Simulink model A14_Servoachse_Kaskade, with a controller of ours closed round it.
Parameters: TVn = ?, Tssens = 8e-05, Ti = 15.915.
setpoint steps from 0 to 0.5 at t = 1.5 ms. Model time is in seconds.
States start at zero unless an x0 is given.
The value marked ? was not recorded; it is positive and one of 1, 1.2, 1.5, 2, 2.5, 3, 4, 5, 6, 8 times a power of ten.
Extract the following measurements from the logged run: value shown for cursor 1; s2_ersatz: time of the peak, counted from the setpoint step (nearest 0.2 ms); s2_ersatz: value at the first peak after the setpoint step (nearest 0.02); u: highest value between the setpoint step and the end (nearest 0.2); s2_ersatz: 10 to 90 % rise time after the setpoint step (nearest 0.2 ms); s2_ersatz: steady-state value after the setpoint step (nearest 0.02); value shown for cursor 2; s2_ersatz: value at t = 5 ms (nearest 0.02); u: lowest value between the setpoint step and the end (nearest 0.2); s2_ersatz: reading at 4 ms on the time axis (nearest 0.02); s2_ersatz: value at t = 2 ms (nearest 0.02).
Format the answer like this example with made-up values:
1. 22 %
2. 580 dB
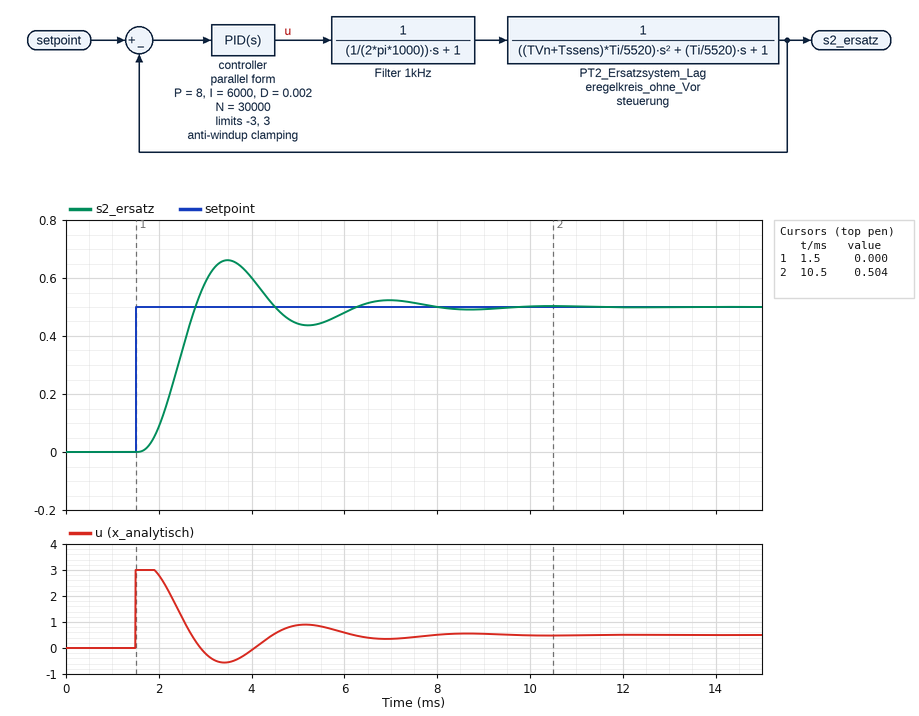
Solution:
1. 0.000
2. 2.0 ms
3. 0.66
4. 3.0
5. 0.8 ms
6. 0.50
7. 0.504
8. 0.44
9. -0.6
10. 0.60
11. 0.08
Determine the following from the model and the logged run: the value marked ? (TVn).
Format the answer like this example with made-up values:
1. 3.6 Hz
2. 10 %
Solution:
1. 0.0006
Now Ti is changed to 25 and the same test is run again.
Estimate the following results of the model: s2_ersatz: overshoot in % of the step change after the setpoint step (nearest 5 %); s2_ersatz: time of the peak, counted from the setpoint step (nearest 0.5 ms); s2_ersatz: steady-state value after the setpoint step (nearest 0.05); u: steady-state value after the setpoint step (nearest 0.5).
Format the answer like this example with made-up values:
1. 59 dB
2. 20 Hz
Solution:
1. 35 %
2. 2.5 ms
3. 0.50
4. 0.5
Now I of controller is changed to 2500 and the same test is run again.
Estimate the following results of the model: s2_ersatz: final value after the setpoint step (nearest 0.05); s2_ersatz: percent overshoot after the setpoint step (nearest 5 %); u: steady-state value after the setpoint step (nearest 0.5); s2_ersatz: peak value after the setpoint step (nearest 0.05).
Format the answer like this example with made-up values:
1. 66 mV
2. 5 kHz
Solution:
1. 0.50
2. 15 %
3. 0.5
4. 0.60
